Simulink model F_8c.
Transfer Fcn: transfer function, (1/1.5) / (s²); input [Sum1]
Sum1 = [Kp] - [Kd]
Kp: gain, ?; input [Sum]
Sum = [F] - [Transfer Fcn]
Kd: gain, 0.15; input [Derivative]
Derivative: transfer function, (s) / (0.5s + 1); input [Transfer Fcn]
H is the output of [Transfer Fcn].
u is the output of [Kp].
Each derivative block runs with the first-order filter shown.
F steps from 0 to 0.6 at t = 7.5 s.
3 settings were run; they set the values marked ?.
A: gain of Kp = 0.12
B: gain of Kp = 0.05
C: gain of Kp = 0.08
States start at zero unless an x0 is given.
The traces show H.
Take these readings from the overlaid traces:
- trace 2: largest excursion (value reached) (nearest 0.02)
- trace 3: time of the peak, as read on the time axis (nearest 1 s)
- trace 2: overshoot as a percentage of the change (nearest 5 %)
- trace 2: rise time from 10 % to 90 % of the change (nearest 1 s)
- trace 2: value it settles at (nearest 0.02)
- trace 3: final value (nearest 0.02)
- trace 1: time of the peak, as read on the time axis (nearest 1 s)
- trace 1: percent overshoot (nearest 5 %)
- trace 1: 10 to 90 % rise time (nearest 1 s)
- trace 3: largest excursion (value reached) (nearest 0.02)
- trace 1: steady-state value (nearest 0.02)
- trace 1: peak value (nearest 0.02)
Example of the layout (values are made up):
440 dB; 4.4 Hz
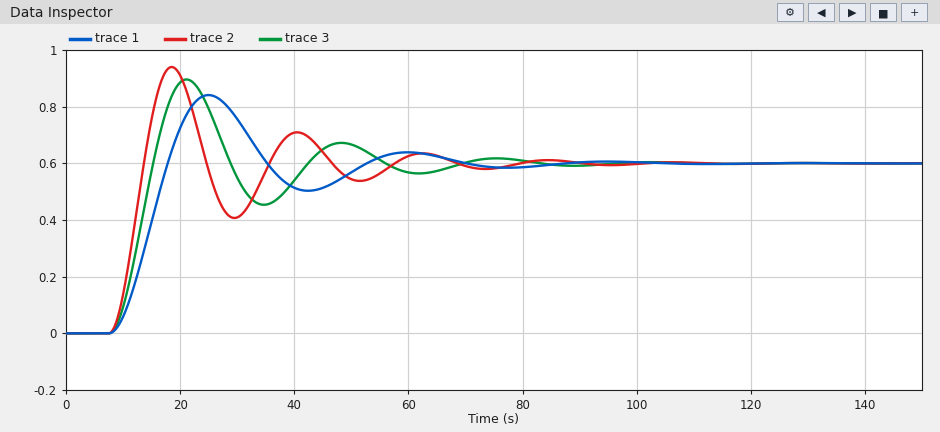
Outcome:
0.94; 21 s; 55 %; 4 s; 0.60; 0.60; 25 s; 40 %; 7 s; 0.90; 0.60; 0.84
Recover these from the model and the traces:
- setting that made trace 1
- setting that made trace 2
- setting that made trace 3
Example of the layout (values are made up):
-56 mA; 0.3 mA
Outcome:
B; A; C
